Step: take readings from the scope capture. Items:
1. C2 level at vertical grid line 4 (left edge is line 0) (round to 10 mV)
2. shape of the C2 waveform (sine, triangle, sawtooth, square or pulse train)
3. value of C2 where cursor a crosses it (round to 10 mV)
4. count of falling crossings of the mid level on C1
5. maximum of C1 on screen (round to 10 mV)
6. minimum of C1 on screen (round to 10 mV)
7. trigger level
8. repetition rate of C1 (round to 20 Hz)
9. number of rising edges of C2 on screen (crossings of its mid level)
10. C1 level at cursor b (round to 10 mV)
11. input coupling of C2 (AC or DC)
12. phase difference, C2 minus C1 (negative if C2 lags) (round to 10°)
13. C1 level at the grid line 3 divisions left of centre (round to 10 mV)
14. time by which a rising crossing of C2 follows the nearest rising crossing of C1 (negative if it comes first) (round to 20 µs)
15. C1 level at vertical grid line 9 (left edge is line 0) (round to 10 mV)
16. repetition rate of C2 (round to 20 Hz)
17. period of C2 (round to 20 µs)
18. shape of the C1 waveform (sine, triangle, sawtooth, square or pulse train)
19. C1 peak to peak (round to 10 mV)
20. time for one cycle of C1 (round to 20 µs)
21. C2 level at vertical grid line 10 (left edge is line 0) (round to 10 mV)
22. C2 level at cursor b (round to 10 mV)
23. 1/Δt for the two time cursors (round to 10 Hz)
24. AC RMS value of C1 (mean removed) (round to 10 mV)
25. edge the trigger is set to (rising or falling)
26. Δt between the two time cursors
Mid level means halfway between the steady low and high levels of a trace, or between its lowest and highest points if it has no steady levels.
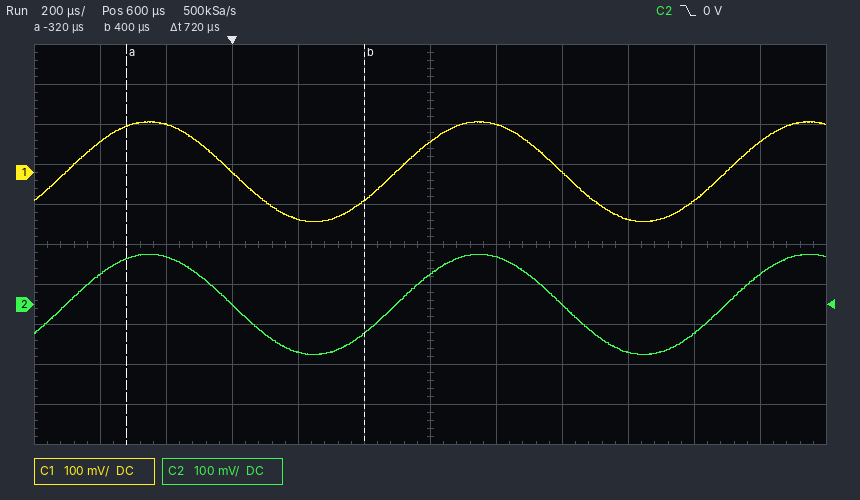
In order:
-120 mV
sine
110 mV
2
130 mV
-120 mV
0 V
1.00 kHz
3
-70 mV
DC
0°
0 mV
0 µs
-120 mV
1.00 kHz
1.00 ms
sine
250 mV
1.00 ms
-70 mV
-70 mV
1.39 kHz
90 mV
falling
720 µs
